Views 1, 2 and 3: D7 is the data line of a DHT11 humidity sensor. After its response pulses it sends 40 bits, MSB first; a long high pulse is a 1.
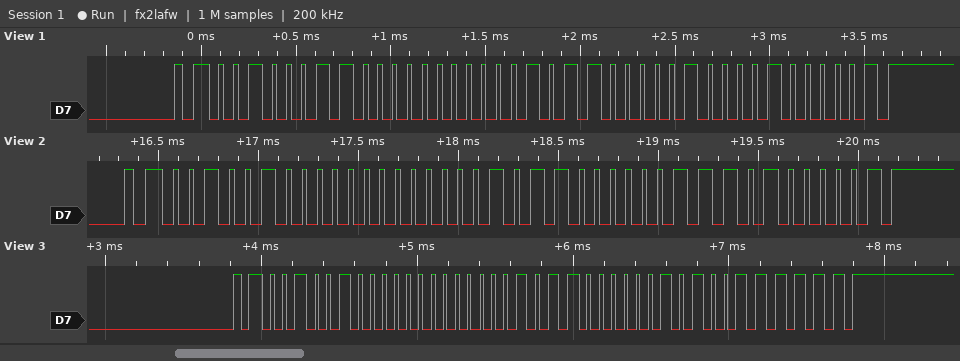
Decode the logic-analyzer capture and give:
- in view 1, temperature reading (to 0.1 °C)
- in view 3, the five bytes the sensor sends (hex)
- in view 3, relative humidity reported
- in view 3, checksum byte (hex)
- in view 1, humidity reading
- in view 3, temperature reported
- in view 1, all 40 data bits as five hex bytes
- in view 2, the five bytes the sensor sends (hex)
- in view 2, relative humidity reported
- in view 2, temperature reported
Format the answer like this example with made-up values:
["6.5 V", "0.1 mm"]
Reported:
["22.8 °C", "24 00 16 05 3F", "36 %", "0x3F", "35 %", "22.5 °C", "23 00 16 08 41", "24 00 16 07 41", "36 %", "22.7 °C"]
